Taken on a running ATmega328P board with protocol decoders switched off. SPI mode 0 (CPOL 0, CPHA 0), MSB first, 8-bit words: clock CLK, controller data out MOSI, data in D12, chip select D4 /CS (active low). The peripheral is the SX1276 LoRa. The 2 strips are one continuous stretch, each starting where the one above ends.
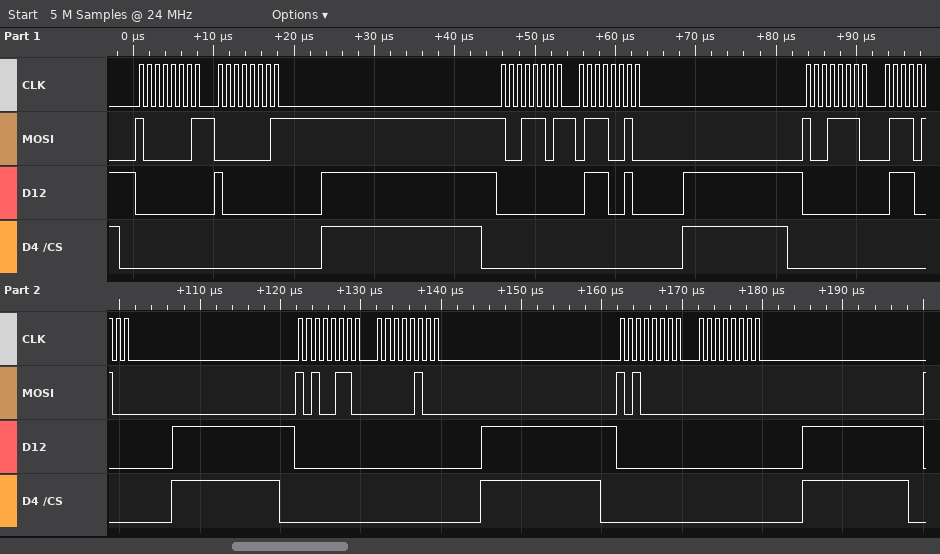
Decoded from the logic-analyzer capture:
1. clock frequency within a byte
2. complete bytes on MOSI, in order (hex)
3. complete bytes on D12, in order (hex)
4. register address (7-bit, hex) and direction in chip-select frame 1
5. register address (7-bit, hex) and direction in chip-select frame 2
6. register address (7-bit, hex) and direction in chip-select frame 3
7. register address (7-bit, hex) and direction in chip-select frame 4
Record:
1 MHz
0x81 0x01 0x9D 0x72 0x9E 0x74 0xA6 0x04 0xA0 0x00
0x00 0x80 0x00 0x72 0x00 0x70 0x00 0x00 0x00 0x00
0x01 write
0x1D write
0x1E write
0x26 write
